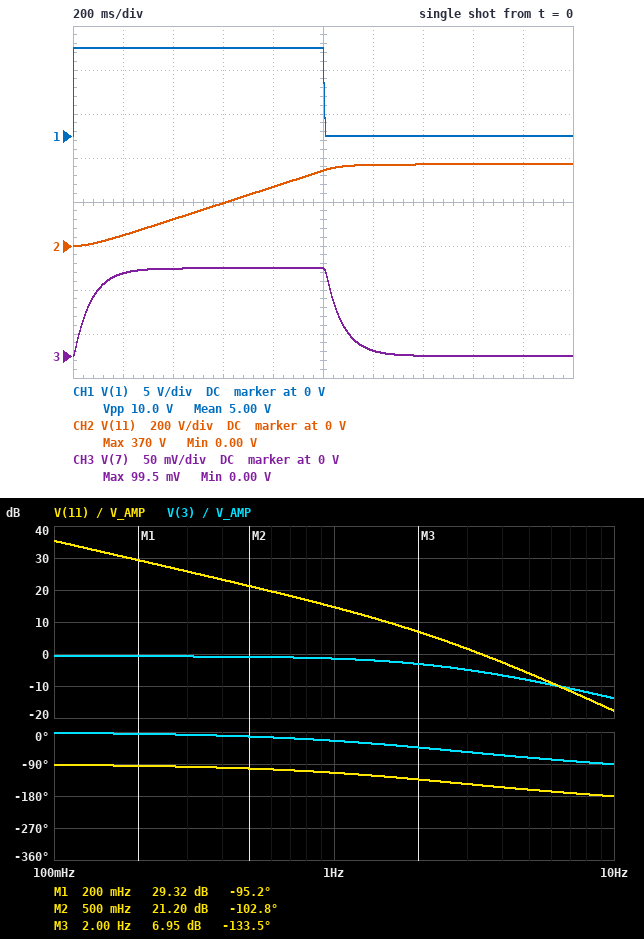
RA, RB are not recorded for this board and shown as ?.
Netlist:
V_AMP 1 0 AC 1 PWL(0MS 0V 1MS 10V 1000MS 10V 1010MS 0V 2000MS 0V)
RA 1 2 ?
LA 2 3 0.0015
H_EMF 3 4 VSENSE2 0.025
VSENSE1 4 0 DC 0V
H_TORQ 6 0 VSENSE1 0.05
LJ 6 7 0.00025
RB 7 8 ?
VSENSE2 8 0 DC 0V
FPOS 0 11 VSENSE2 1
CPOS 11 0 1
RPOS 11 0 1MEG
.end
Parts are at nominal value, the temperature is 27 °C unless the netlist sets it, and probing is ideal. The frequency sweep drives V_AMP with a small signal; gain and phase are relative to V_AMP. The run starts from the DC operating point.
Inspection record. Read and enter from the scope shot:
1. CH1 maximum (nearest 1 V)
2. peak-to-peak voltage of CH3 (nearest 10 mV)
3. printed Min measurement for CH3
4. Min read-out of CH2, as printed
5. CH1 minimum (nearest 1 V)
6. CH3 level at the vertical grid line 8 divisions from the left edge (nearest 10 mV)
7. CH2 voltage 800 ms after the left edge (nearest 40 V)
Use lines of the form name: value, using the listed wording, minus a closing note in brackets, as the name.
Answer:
CH1 maximum: 10 V
peak-to-peak voltage of CH3: 100 mV
printed Min measurement for CH3: 0.00 V
Min read-out of CH2, as printed: 0.00 V
CH1 minimum: 0 V
CH3 level at the vertical grid line 8 divisions from the left edge: 0 V
CH2 voltage 800 ms after the left edge: 280 V
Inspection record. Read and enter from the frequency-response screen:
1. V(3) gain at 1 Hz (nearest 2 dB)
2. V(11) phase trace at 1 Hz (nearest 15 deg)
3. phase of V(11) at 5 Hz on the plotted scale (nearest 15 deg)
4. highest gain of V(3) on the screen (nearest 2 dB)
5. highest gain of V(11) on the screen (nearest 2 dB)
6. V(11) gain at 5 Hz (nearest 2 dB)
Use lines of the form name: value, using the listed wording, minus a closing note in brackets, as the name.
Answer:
V(3) gain at 1 Hz: -2 dB
V(11) phase trace at 1 Hz: -120 deg
phase of V(11) at 5 Hz on the plotted scale: -165 deg
highest gain of V(3) on the screen: 0 dB
highest gain of V(11) on the screen: 36 dB
V(11) gain at 5 Hz: -6 dB
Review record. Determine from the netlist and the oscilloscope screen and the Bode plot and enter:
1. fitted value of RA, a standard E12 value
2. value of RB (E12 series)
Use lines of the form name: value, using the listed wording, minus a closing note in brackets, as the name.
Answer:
fitted value of RA, a standard E12 value: 0.39 Ω
value of RB: 270 µΩ
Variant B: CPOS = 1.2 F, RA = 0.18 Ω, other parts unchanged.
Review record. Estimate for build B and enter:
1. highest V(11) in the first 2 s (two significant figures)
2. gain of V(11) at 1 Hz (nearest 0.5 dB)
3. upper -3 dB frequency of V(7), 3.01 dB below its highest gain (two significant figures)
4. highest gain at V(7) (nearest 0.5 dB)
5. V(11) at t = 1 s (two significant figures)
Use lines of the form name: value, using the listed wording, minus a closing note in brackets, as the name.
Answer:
highest V(11) in the first 2 s: 320 V
gain of V(11) at 1 Hz: 14.0 dB
upper -3 dB frequency of V(7), 3.01 dB below its highest gain: 5.8 Hz
highest gain at V(7): -39.5 dB
V(11) at t = 1 s: 310 V
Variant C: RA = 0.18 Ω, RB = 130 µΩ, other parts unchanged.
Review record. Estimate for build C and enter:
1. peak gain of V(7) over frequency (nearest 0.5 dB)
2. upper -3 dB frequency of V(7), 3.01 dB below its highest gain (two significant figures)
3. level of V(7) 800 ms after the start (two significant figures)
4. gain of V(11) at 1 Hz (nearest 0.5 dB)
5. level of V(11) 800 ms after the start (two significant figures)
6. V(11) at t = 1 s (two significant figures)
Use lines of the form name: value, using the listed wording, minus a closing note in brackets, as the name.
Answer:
peak gain of V(7) over frequency: -46.0 dB
upper -3 dB frequency of V(7), 3.01 dB below its highest gain: 5.7 Hz
level of V(7) 800 ms after the start: 51 mV
gain of V(11) at 1 Hz: 16.0 dB
level of V(11) 800 ms after the start: 300 V
V(11) at t = 1 s: 380 V
